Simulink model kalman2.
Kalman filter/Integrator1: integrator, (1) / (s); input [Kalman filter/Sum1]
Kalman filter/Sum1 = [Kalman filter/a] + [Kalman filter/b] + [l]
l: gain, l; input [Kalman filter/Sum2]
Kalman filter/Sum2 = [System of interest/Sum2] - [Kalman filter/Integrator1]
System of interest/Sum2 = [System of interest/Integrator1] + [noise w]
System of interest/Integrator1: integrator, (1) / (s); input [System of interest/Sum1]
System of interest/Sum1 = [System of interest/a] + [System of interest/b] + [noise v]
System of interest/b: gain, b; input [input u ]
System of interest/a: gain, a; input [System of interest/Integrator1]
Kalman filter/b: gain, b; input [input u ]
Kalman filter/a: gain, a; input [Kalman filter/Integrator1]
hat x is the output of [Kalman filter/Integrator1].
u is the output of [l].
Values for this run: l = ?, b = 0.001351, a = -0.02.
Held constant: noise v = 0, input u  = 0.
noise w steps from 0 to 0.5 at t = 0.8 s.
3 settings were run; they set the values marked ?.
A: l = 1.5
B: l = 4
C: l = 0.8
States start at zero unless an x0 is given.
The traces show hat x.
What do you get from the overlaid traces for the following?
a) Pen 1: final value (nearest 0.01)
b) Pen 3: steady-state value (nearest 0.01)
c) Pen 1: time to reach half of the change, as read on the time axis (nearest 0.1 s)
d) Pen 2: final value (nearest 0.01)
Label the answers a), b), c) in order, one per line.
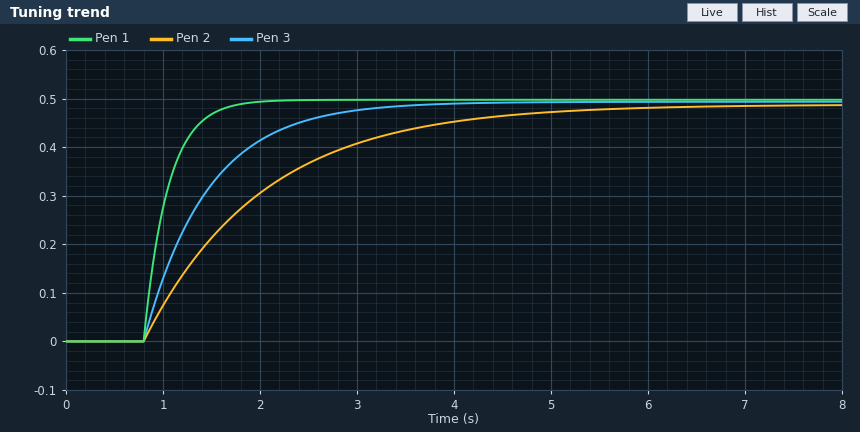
a) 0.50
b) 0.49
c) 1.0 s
d) 0.49
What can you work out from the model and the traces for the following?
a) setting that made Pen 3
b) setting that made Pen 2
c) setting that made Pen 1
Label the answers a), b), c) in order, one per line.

a) A
b) C
c) B
